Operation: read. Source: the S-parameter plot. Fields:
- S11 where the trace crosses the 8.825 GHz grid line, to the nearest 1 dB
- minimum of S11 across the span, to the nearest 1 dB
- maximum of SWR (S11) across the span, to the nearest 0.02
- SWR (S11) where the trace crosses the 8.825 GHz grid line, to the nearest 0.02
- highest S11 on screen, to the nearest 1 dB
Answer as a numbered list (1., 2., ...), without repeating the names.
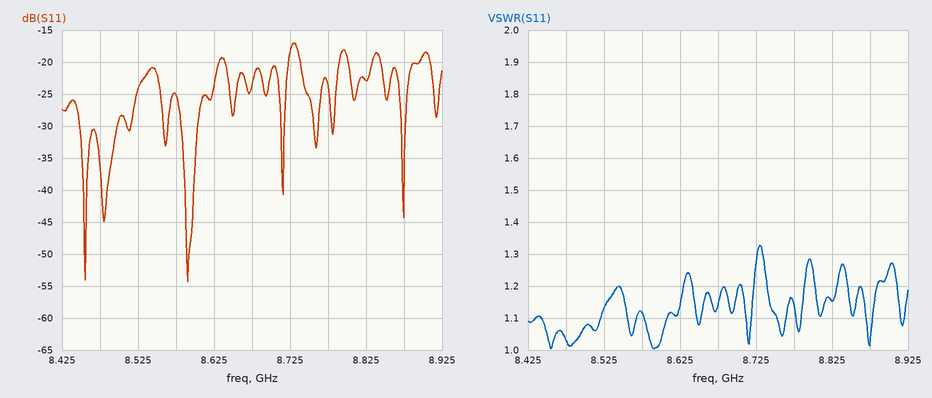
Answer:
1. -23 dB
2. -54 dB
3. 1.32
4. 1.16
5. -17 dB
